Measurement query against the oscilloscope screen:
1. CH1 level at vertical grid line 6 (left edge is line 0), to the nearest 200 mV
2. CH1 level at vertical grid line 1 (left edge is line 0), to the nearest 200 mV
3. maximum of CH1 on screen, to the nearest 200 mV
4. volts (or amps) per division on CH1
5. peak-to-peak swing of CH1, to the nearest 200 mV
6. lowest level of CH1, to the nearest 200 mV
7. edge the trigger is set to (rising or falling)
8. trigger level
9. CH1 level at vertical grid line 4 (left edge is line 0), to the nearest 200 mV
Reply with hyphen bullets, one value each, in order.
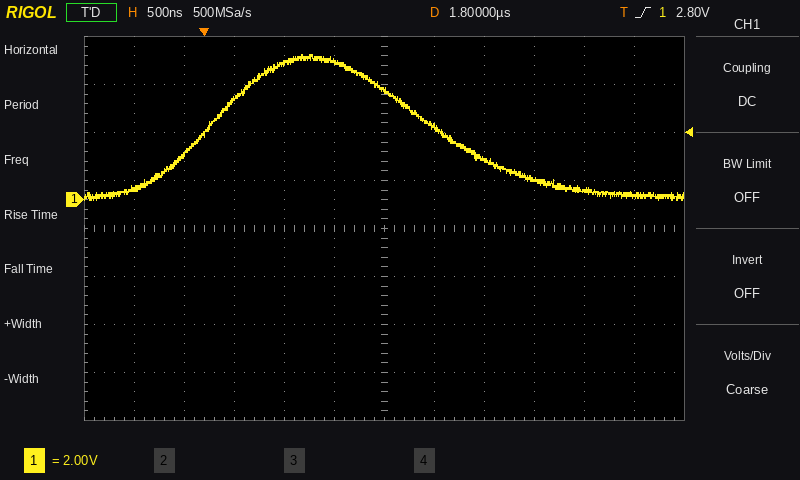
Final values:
- 4.6 V
- 400 mV
- 6.0 V
- 2 V
- 6.0 V
- 0.0 V
- rising
- 2.80 V
- 5.6 V
